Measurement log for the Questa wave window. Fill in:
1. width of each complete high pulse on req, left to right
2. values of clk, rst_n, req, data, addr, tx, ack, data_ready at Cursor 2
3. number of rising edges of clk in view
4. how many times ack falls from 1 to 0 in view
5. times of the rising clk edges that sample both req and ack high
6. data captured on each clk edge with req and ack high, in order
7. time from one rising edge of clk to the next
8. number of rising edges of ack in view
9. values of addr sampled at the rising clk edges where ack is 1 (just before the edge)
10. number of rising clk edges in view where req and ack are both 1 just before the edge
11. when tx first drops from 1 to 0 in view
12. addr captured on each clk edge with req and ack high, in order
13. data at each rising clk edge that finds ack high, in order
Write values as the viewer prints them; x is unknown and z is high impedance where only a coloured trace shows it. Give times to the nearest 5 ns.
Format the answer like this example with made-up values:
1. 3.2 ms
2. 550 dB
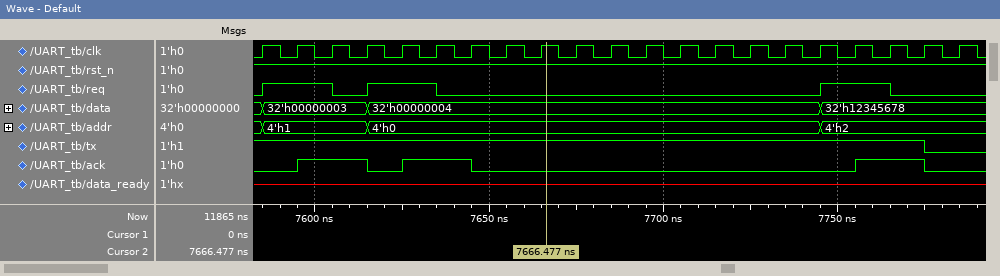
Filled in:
1. 20 ns, 20 ns, 20 ns
2. clk=1, rst_n=1, req=0, data=32'h00000004, addr=4'h0, tx=1, ack=0, data_ready=x
3. 21
4. 3
5. 7605 ns, 7635 ns, 7765 ns
6. 32'h00000003, 32'h00000004, 32'h12345678
7. 10 ns
8. 3
9. 4'h1, 4'h1, 4'h0, 4'h0, 4'h2, 4'h2
10. 3
11. 7775 ns
12. 4'h1, 4'h0, 4'h2
13. 32'h00000003, 32'h00000003, 32'h00000004, 32'h00000004, 32'h12345678, 32'h12345678
